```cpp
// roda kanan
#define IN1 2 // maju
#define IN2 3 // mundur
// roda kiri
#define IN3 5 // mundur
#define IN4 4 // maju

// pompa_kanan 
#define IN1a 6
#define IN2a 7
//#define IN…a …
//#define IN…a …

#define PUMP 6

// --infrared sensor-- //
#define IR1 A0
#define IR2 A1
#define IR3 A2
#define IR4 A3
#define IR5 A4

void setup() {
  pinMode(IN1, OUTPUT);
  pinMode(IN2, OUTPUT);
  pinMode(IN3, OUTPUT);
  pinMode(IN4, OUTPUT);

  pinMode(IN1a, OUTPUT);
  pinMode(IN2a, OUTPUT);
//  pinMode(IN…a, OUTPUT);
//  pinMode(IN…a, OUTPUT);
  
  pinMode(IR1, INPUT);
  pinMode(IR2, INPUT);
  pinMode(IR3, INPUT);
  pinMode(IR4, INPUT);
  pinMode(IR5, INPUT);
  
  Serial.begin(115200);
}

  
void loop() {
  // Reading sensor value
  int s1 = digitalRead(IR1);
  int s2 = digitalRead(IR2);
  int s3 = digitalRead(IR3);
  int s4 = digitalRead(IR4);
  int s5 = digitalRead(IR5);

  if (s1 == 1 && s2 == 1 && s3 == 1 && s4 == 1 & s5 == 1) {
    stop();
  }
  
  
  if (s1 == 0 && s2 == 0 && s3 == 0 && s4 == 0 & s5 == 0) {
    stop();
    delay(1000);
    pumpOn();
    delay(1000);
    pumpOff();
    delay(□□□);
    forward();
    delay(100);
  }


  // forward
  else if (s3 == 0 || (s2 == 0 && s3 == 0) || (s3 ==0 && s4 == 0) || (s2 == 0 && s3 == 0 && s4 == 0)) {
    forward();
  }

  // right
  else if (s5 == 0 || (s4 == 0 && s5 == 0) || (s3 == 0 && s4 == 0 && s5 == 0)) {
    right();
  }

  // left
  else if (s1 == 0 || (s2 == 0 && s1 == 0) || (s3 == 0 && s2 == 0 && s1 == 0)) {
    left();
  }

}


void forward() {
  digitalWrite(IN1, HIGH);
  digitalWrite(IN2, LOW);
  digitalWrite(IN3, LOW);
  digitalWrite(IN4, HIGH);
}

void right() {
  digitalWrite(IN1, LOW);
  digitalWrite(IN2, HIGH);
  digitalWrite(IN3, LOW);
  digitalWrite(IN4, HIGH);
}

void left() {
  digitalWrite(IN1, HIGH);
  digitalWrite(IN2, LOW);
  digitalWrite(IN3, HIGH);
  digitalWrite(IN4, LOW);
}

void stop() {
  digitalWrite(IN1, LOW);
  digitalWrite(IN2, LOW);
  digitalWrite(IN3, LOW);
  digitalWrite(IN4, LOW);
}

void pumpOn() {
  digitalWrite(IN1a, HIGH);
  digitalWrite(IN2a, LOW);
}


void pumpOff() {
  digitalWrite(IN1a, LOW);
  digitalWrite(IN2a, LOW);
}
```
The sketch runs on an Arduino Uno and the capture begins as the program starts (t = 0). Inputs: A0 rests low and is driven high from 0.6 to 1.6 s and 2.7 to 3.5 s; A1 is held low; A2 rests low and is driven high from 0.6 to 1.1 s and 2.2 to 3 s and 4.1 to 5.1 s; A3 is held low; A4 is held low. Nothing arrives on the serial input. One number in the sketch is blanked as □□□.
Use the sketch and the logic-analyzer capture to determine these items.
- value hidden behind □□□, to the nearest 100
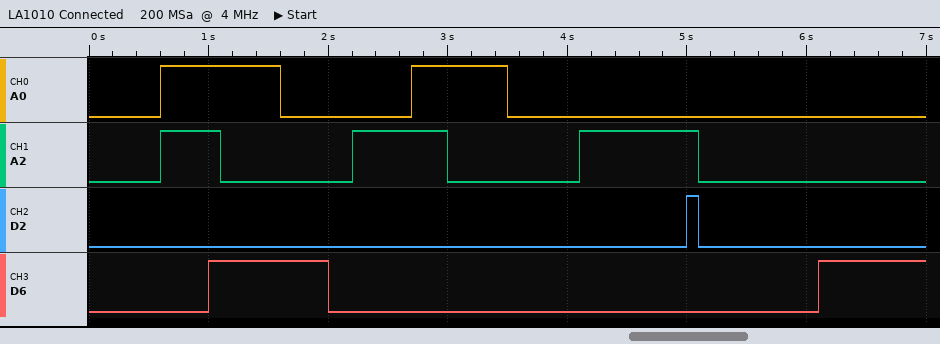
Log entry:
3000
